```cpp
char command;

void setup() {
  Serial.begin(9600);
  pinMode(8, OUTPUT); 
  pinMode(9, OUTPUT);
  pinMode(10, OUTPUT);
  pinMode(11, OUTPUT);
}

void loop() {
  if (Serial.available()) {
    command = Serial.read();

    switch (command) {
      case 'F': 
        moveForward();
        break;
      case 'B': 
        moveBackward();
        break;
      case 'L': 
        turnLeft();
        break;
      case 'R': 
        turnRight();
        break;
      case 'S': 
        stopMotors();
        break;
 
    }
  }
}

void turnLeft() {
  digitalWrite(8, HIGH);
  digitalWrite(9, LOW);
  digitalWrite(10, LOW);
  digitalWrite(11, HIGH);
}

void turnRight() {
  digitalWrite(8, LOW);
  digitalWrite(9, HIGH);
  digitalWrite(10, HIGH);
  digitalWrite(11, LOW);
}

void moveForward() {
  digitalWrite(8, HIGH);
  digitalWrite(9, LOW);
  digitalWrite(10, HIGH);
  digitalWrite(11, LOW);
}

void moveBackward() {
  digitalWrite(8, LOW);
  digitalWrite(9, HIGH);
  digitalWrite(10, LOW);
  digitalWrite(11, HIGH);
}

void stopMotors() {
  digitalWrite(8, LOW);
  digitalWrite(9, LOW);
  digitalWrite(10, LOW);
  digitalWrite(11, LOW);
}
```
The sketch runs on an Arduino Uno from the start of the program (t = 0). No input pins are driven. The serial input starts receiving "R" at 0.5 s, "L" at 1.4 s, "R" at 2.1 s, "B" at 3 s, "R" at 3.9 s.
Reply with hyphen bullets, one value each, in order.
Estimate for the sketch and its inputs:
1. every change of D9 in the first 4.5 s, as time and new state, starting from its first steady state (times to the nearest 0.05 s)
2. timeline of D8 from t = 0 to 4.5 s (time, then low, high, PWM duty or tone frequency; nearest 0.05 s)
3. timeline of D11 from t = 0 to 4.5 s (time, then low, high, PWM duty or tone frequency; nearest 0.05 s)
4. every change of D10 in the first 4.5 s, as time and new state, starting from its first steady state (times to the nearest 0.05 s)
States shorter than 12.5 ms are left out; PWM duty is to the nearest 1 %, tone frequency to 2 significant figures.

- 0 s low; 0.5 s high; 1.4 s low; 2.1 s high
- 0 s low; 1.4 s high; 2.1 s low
- 0 s low; 1.4 s high; 2.1 s low; 3 s high; 3.9 s low
- 0 s low; 0.5 s high; 1.4 s low; 2.1 s high; 3 s low; 3.9 s high
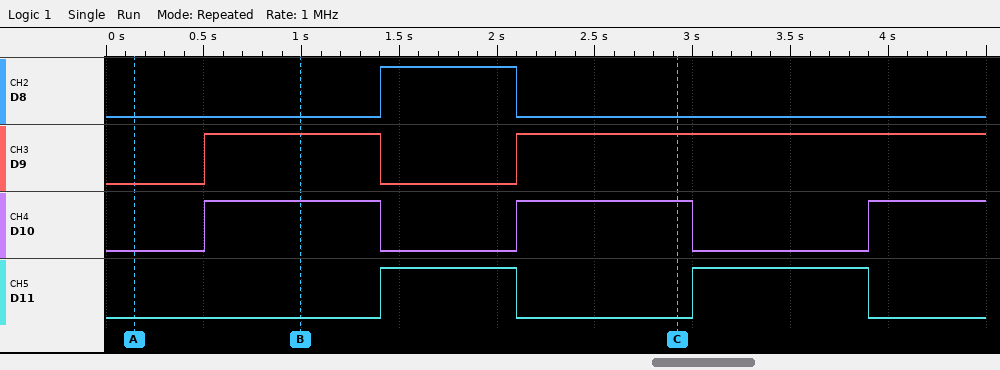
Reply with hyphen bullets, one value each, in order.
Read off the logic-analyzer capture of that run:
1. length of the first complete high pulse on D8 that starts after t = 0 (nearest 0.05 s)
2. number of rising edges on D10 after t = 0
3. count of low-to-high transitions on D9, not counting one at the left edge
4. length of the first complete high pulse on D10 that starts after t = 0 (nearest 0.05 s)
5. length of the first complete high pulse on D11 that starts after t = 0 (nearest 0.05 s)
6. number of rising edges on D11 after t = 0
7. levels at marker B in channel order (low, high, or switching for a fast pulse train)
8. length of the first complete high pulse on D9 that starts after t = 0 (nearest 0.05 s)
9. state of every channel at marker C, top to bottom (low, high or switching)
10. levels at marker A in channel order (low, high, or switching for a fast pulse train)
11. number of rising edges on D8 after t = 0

- 0.70 s
- 3
- 2
- 0.90 s
- 0.70 s
- 2
- D8 low, D9 high, D10 high, D11 low
- 0.90 s
- D8 low, D9 high, D10 high, D11 low
- D8 low, D9 low, D10 low, D11 low
- 1
